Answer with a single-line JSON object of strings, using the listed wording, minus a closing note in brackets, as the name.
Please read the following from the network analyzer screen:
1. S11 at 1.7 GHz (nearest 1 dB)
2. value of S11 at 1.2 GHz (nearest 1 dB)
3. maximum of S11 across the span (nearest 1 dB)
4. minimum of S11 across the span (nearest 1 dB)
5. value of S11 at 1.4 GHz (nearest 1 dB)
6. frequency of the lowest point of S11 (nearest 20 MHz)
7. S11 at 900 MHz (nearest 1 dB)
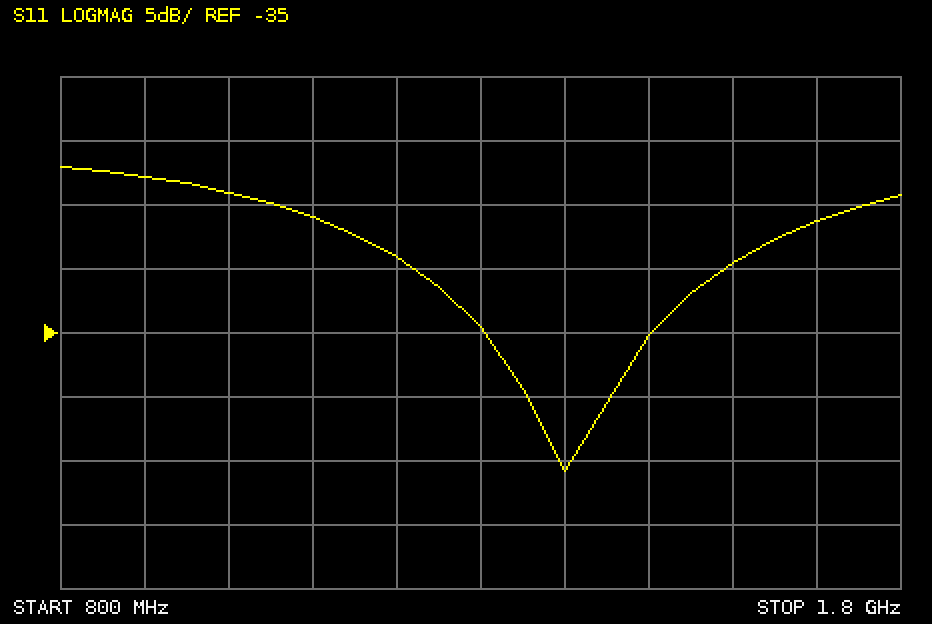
{"S11 at 1.7 GHz": "-26 dB", "value of S11 at 1.2 GHz": "-29 dB", "maximum of S11 across the span": "-22 dB", "minimum of S11 across the span": "-46 dB", "value of S11 at 1.4 GHz": "-46 dB", "frequency of the lowest point of S11": "1.40 GHz", "S11 at 900 MHz": "-23 dB"}
